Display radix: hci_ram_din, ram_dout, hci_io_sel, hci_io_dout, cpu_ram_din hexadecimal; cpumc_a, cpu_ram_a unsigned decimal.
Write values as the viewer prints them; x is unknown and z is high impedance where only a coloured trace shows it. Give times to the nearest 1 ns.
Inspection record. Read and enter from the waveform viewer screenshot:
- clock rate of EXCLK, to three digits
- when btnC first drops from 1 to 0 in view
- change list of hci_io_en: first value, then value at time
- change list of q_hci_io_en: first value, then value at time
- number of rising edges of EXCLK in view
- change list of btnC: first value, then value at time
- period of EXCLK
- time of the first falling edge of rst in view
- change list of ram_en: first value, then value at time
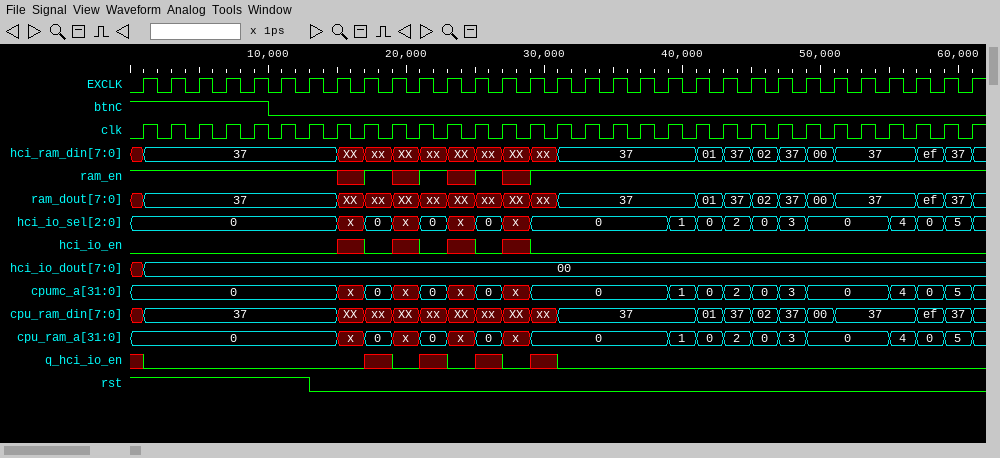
500 MHz
10 ns
0, x at 15 ns, 0 at 17 ns, x at 19 ns, 0 at 21 ns, x at 23 ns, 0 at 25 ns, x at 27 ns, 0 at 29 ns
x, 0 at 1 ns, x at 17 ns, 0 at 19 ns, x at 21 ns, 0 at 23 ns, x at 25 ns, 0 at 27 ns, x at 29 ns, 0 at 31 ns
31
1, 0 at 10 ns
2 ns
13 ns
1, x at 15 ns, 1 at 17 ns, x at 19 ns, 1 at 21 ns, x at 23 ns, 1 at 25 ns, x at 27 ns, 1 at 29 ns
